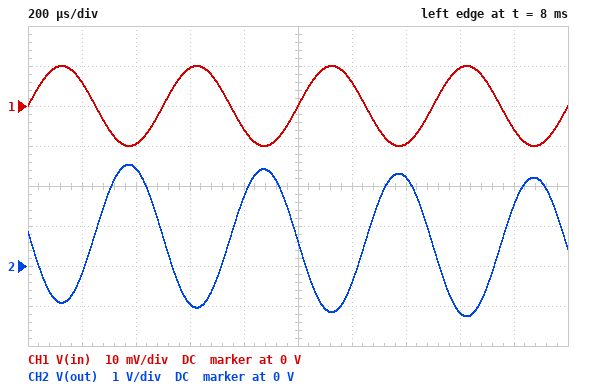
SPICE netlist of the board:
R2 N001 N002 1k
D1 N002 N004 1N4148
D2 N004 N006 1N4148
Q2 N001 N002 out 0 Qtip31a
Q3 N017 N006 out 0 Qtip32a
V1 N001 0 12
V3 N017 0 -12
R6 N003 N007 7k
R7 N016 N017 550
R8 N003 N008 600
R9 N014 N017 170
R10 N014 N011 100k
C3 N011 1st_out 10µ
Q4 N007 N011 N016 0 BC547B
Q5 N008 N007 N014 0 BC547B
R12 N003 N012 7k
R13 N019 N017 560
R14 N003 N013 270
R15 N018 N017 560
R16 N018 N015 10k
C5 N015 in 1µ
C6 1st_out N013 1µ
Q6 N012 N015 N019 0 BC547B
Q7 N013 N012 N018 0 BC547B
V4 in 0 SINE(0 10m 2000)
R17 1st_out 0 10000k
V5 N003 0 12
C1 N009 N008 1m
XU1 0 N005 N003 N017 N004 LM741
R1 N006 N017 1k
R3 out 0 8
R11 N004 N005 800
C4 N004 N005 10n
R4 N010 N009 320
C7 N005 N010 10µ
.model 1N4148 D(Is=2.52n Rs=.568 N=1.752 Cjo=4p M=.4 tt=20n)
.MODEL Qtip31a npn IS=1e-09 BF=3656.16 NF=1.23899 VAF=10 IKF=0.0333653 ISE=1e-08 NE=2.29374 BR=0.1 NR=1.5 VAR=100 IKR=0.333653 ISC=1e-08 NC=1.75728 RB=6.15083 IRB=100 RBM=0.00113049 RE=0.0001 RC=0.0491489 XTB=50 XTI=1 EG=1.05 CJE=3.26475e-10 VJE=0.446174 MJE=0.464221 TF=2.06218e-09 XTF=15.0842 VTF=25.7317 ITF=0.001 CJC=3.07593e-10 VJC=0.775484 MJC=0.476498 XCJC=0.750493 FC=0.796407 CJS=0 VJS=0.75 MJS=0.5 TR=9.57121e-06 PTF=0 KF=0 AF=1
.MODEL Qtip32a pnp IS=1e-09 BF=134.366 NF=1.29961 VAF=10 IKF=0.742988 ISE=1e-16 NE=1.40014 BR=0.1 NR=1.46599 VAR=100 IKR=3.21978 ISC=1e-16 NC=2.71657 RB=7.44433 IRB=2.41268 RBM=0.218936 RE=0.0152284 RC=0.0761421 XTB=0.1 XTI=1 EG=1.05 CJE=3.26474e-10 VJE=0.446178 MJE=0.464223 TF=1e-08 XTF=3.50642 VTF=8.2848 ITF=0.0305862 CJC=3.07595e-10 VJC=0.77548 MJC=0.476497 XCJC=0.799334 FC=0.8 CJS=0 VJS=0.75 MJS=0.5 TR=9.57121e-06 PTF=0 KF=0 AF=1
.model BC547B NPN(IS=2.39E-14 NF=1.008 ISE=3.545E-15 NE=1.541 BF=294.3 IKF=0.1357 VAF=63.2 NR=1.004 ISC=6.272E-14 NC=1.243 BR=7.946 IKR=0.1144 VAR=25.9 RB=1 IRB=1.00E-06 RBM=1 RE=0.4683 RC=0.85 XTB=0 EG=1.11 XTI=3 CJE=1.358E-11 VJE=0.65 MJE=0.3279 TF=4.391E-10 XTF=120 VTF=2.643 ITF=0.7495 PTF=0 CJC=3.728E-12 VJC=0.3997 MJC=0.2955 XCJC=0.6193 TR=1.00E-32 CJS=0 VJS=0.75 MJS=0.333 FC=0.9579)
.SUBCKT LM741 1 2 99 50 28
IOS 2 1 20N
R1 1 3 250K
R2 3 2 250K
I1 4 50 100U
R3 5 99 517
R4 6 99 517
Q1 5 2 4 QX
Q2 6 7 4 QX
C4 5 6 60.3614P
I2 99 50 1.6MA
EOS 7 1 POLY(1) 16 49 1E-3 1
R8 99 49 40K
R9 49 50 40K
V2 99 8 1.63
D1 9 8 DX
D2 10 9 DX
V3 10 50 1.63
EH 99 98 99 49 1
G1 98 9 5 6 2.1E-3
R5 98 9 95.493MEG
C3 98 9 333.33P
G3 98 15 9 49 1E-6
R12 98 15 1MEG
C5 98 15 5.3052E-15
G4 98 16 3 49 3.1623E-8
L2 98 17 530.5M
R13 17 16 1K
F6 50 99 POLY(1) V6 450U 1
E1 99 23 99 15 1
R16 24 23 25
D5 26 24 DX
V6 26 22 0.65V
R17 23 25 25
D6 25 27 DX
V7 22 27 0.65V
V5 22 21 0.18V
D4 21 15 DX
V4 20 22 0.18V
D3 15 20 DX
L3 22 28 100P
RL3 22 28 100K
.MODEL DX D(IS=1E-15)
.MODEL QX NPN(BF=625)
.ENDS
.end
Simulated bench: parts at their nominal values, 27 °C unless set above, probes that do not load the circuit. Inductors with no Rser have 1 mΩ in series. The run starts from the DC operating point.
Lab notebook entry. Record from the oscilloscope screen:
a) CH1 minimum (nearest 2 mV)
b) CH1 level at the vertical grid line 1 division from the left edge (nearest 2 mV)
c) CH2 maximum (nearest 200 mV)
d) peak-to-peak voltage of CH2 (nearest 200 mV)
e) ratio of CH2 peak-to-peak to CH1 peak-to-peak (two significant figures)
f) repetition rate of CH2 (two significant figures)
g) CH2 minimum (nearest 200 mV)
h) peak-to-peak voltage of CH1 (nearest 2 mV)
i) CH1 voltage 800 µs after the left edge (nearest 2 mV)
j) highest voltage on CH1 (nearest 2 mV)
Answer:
-10 mV
6 mV
2.6 V
3.8 V
190
2.0 kHz
-1.2 V
20 mV
-6 mV
10 mV
